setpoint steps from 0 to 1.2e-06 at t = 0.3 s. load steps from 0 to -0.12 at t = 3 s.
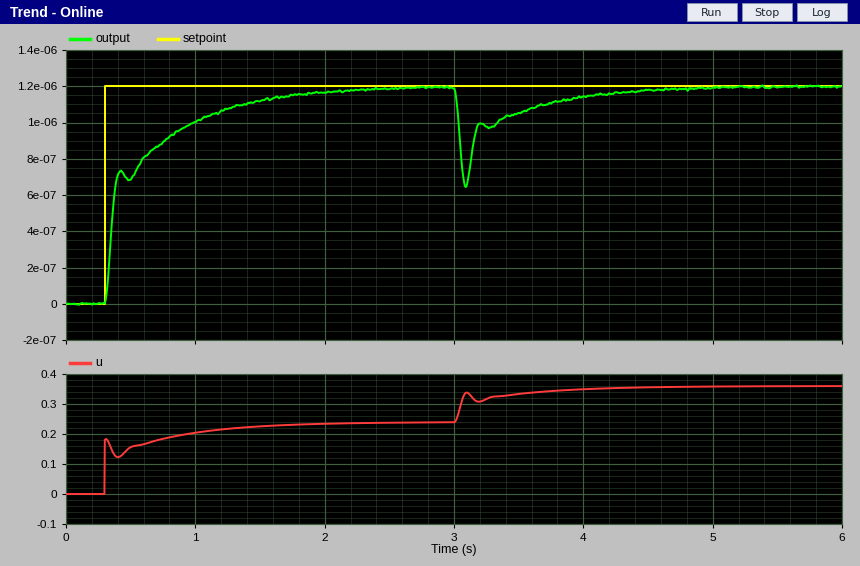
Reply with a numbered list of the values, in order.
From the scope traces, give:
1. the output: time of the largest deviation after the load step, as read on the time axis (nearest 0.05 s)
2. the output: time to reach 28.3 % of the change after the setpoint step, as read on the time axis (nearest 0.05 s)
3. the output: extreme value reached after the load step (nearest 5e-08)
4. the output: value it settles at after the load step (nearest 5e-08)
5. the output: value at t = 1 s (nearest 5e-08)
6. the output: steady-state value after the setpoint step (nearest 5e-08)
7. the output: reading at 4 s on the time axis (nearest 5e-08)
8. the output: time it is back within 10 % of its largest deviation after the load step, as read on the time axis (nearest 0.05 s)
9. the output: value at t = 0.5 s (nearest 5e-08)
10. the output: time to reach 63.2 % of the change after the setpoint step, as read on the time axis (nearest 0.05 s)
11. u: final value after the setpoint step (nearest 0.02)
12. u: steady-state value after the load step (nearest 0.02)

1. 3.10 s
2. 0.35 s
3. 0.00000065
4. 0.00000120
5. 0.00000100
6. 0.00000120
7. 0.00000115
8. 4.05 s
9. 0.00000070
10. 0.55 s
11. 0.24
12. 0.36
